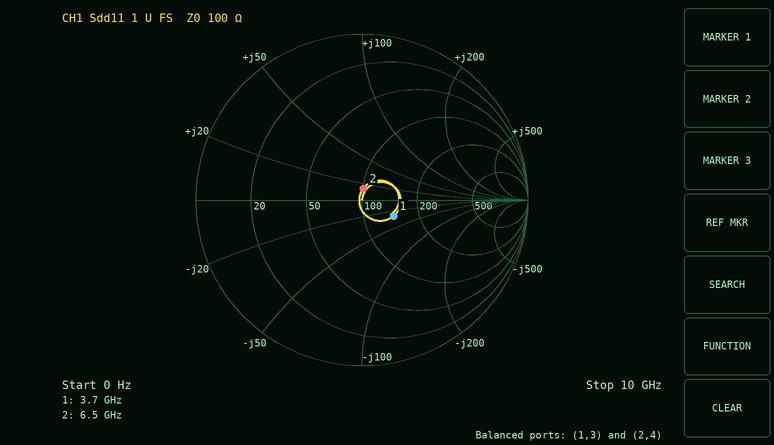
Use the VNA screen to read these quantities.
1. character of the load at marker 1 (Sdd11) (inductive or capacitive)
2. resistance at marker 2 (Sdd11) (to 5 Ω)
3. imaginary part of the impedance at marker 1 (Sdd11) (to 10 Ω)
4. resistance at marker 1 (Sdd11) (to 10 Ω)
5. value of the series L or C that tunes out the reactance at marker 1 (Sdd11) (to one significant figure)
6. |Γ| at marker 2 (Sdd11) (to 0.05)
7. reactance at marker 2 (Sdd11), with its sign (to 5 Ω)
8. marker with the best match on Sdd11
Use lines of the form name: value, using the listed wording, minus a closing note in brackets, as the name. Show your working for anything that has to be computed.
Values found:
character of the load at marker 1 (Sdd11): capacitive
resistance at marker 2 (Sdd11): 100 Ω
imaginary part of the impedance at marker 1 (Sdd11): -30 Ω
resistance at marker 1 (Sdd11): 140 Ω
value of the series L or C that tunes out the reactance at marker 1 (Sdd11): L = 30 Ω/(2π × 3.7 GHz) ≈ 1 nH
|Γ| at marker 2 (Sdd11): 0.05
reactance at marker 2 (Sdd11), with its sign: +15 Ω
marker with the best match on Sdd11: marker 2
